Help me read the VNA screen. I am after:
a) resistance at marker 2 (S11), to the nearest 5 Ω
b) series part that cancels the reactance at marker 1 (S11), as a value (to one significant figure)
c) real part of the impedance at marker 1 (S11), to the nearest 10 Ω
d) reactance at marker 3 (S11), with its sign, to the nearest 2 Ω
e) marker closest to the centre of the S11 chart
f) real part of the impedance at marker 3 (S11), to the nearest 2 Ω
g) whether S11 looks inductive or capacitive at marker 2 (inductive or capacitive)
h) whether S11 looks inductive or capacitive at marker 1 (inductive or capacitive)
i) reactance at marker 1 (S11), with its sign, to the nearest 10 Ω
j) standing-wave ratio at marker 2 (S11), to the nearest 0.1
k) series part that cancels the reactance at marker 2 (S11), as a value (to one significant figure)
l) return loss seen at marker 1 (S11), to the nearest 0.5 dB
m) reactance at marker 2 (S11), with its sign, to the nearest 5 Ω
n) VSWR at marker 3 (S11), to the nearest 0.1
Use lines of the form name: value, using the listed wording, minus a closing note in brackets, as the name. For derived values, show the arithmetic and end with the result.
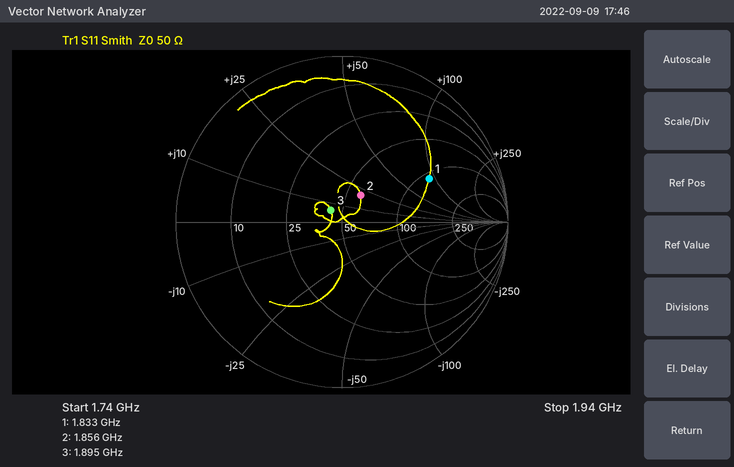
resistance at marker 2 (S11), to the nearest 5 Ω: 60 Ω
series part that cancels the reactance at marker 1 (S11), as a value: C = 1/(2π × 1.833 GHz × 90 Ω) ≈ 1.0 pF
real part of the impedance at marker 1 (S11), to the nearest 10 Ω: 110 Ω
reactance at marker 3 (S11), with its sign, to the nearest 2 Ω: +6 Ω
marker closest to the centre of the S11 chart: marker 3
real part of the impedance at marker 3 (S11), to the nearest 2 Ω: 44 Ω
whether S11 looks inductive or capacitive at marker 2: inductive
whether S11 looks inductive or capacitive at marker 1: inductive
reactance at marker 1 (S11), with its sign, to the nearest 10 Ω: +90 Ω
standing-wave ratio at marker 2 (S11), to the nearest 0.1: 1.5
series part that cancels the reactance at marker 2 (S11), as a value: C = 1/(2π × 1.856 GHz × 20 Ω) ≈ 4 pF
return loss seen at marker 1 (S11), to the nearest 0.5 dB: 4.5 dB
reactance at marker 2 (S11), with its sign, to the nearest 5 Ω: +20 Ω
VSWR at marker 3 (S11), to the nearest 0.1: 1.2
